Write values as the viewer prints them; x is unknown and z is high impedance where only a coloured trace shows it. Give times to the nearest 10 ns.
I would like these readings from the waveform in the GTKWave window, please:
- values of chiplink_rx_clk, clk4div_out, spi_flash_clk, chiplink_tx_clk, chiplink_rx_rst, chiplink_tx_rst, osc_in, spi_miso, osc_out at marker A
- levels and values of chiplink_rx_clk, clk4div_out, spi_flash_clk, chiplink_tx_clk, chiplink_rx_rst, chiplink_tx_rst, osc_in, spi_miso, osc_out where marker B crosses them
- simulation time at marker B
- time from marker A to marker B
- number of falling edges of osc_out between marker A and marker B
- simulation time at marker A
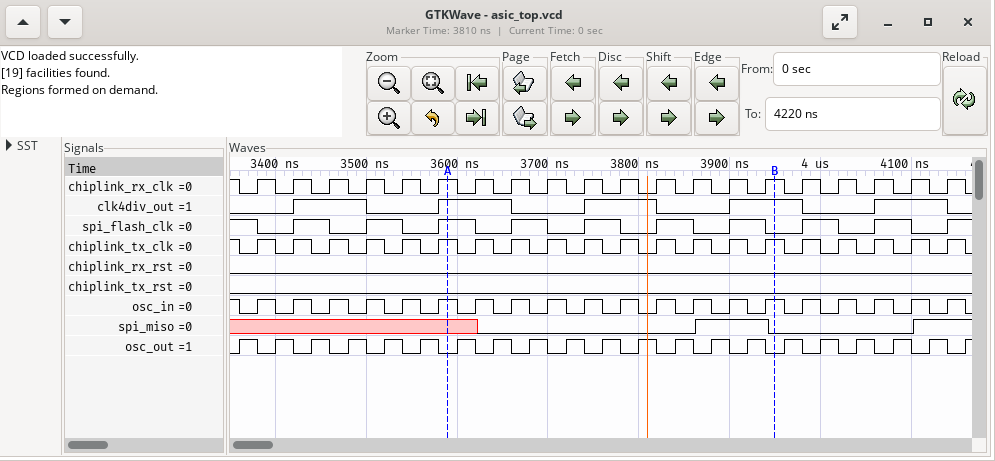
chiplink_rx_clk=1, clk4div_out=1, spi_flash_clk=1, chiplink_tx_clk=1, chiplink_rx_rst=0, chiplink_tx_rst=0, osc_in=1, spi_miso=x, osc_out=0
chiplink_rx_clk=1, clk4div_out=1, spi_flash_clk=0, chiplink_tx_clk=1, chiplink_rx_rst=0, chiplink_tx_rst=0, osc_in=1, spi_miso=0, osc_out=0
3950 ns
360 ns
9
3590 ns
